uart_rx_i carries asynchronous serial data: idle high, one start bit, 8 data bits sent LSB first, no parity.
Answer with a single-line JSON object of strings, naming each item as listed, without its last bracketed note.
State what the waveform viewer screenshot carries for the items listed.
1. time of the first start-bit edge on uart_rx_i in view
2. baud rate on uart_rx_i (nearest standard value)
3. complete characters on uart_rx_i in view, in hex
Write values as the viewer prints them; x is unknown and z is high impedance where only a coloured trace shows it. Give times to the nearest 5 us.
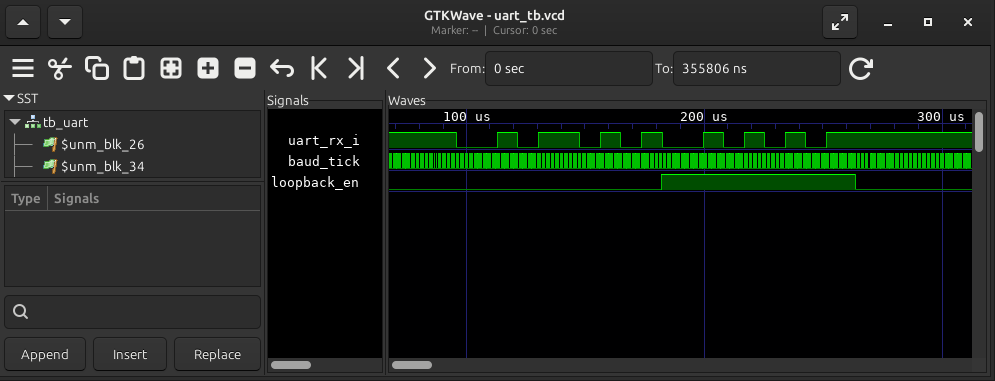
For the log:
{"time of the first start-bit edge on uart_rx_i in view": "95 us", "baud rate on uart_rx_i": "115200 baud", "complete characters on uart_rx_i in view, in hex": "5A, AA"}
